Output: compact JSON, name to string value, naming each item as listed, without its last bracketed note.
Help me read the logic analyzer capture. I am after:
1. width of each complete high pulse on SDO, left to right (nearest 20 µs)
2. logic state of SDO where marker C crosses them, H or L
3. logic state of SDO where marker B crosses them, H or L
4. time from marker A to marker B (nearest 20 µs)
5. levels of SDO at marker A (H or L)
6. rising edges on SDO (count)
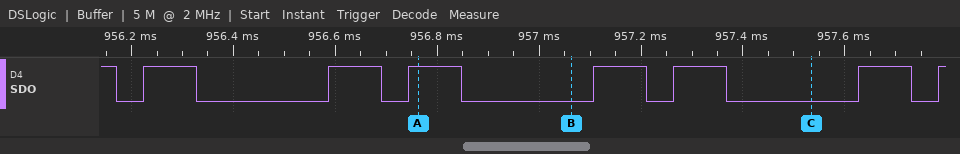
{"width of each complete high pulse on SDO, left to right": "100 µs, 100 µs, 100 µs, 100 µs, 100 µs, 100 µs", "logic state of SDO where marker C crosses them, H or L": "SDO=L", "logic state of SDO where marker B crosses them, H or L": "SDO=L", "time from marker A to marker B": "300 µs", "levels of SDO at marker A": "SDO=H", "rising edges on SDO": "7"}
